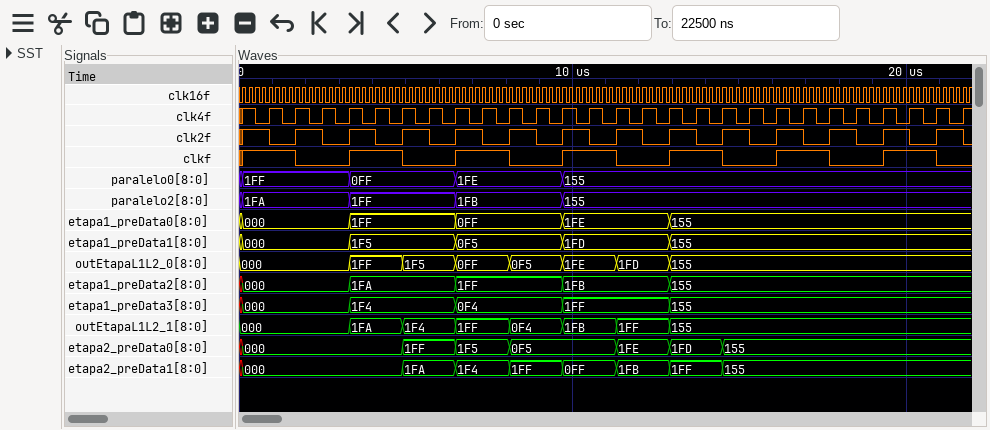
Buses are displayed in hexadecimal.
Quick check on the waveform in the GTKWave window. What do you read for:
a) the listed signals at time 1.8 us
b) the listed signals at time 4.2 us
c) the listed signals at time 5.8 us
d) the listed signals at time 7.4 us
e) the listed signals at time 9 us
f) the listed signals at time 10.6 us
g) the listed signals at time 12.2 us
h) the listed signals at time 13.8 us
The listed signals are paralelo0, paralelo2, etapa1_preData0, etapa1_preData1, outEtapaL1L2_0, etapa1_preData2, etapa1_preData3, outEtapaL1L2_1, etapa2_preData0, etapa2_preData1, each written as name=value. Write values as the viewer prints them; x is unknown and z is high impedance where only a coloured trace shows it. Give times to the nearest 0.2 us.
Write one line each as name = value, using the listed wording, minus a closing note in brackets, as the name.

the listed signals at time 1.8 us = paralelo0=1FF, paralelo2=1FA, etapa1_preData0=000, etapa1_preData1=000, outEtapaL1L2_0=000, etapa1_preData2=000, etapa1_preData3=000, outEtapaL1L2_1=000, etapa2_preData0=000, etapa2_preData1=000
the listed signals at time 4.2 us = paralelo0=0FF, paralelo2=1FF, etapa1_preData0=1FF, etapa1_preData1=1F5, outEtapaL1L2_0=1FF, etapa1_preData2=1FA, etapa1_preData3=1F4, outEtapaL1L2_1=1FA, etapa2_preData0=000, etapa2_preData1=000
the listed signals at time 5.8 us = paralelo0=0FF, paralelo2=1FF, etapa1_preData0=1FF, etapa1_preData1=1F5, outEtapaL1L2_0=1F5, etapa1_preData2=1FA, etapa1_preData3=1F4, outEtapaL1L2_1=1F4, etapa2_preData0=1FF, etapa2_preData1=1FA
the listed signals at time 7.4 us = paralelo0=1FE, paralelo2=1FB, etapa1_preData0=0FF, etapa1_preData1=0F5, outEtapaL1L2_0=0FF, etapa1_preData2=1FF, etapa1_preData3=0F4, outEtapaL1L2_1=1FF, etapa2_preData0=1F5, etapa2_preData1=1F4
the listed signals at time 9 us = paralelo0=1FE, paralelo2=1FB, etapa1_preData0=0FF, etapa1_preData1=0F5, outEtapaL1L2_0=0F5, etapa1_preData2=1FF, etapa1_preData3=0F4, outEtapaL1L2_1=0F4, etapa2_preData0=0F5, etapa2_preData1=1FF
the listed signals at time 10.6 us = paralelo0=155, paralelo2=155, etapa1_preData0=1FE, etapa1_preData1=1FD, outEtapaL1L2_0=1FE, etapa1_preData2=1FB, etapa1_preData3=1FF, outEtapaL1L2_1=1FB, etapa2_preData0=0F5, etapa2_preData1=0FF
the listed signals at time 12.2 us = paralelo0=155, paralelo2=155, etapa1_preData0=1FE, etapa1_preData1=1FD, outEtapaL1L2_0=1FD, etapa1_preData2=1FB, etapa1_preData3=1FF, outEtapaL1L2_1=1FF, etapa2_preData0=1FE, etapa2_preData1=1FB
the listed signals at time 13.8 us = paralelo0=155, paralelo2=155, etapa1_preData0=155, etapa1_preData1=155, outEtapaL1L2_0=155, etapa1_preData2=155, etapa1_preData3=155, outEtapaL1L2_1=155, etapa2_preData0=1FD, etapa2_preData1=1FF
